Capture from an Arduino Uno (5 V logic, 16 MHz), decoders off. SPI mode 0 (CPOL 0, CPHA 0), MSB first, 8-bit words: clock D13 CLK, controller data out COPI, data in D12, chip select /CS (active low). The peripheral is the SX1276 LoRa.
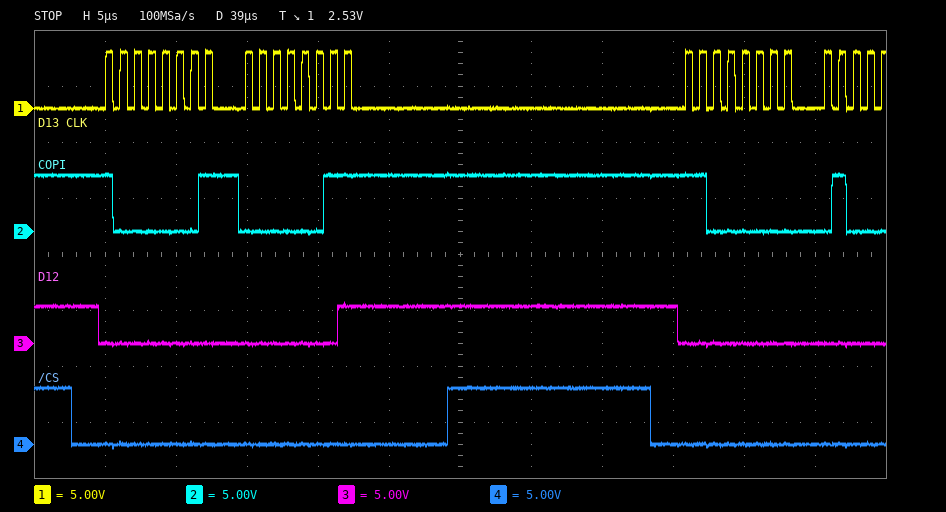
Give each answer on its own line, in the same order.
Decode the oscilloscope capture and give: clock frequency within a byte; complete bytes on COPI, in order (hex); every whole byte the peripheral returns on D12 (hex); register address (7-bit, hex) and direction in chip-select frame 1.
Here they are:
1 MHz
81 03 C0
00 01 00
0x01 write
